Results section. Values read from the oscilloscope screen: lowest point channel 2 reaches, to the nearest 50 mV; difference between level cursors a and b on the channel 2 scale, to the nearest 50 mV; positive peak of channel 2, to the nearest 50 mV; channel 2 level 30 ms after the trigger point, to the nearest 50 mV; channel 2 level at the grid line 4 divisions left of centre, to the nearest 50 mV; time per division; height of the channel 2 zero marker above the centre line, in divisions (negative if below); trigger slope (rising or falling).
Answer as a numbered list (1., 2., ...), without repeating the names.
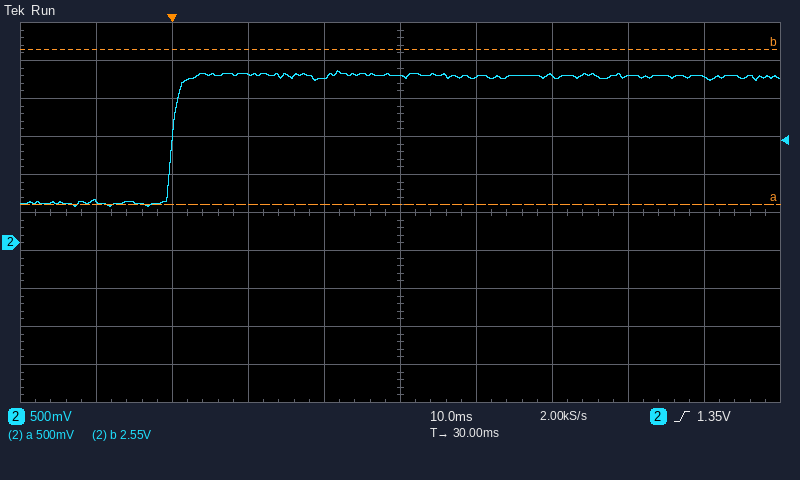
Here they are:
1. 500 mV
2. 2.05 V
3. 2.25 V
4. 2.20 V
5. 550 mV
6. 10 ms
7. -0.8 div
8. rising
